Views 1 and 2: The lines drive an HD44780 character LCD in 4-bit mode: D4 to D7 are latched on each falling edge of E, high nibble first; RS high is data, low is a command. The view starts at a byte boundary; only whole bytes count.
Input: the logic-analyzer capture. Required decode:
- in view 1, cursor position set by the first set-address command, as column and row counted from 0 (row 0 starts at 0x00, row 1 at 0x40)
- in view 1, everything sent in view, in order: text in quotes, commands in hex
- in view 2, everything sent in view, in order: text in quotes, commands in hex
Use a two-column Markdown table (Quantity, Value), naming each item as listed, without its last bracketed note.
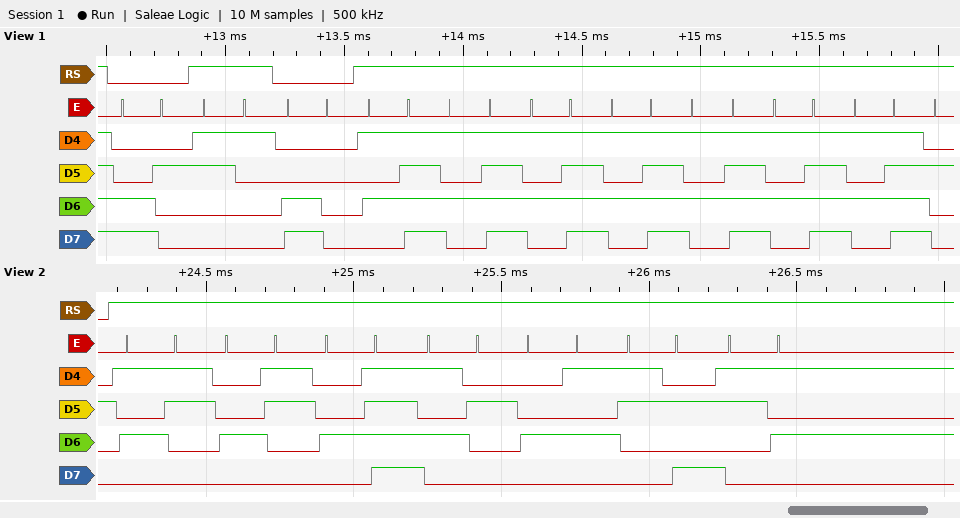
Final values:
| Quantity | Value |
|---|---|
| in view 1, cursor position set by the first set-address command, as column and row counted from 0 | column 2, row 1 |
| in view 1, everything sent in view, in order: text in quotes, commands in hex | 0xC2 "1" 0xC0 "_______" |
| in view 2, everything sent in view, in order: text in quotes, commands in hex | "SCORE:5" |
